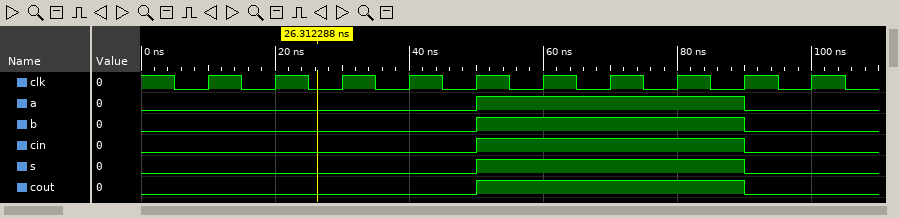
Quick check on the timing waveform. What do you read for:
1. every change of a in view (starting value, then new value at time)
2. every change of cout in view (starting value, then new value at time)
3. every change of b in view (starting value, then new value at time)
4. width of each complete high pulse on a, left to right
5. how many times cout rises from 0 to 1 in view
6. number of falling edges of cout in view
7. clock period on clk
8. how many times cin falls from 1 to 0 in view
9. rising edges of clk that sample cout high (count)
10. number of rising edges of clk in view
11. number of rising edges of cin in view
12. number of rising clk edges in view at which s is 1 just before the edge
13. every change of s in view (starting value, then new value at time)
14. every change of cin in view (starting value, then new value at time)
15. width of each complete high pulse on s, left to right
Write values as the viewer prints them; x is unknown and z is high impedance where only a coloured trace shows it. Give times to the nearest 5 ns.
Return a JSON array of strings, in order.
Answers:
["0, 1 at 50 ns, 0 at 90 ns", "0, 1 at 50 ns, 0 at 90 ns", "0, 1 at 50 ns, 0 at 90 ns", "40 ns", "1", "1", "10 ns", "1", "4", "10", "1", "4", "0, 1 at 50 ns, 0 at 90 ns", "0, 1 at 50 ns, 0 at 90 ns", "40 ns"]
